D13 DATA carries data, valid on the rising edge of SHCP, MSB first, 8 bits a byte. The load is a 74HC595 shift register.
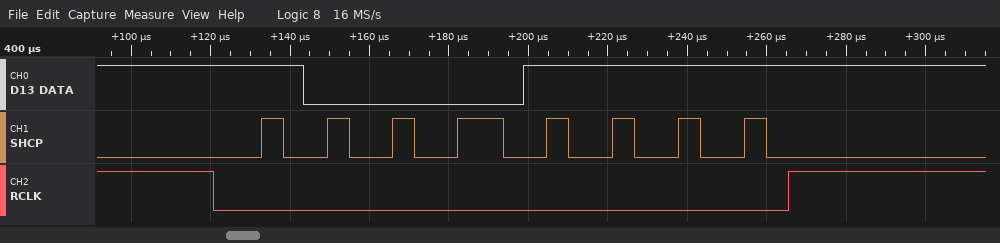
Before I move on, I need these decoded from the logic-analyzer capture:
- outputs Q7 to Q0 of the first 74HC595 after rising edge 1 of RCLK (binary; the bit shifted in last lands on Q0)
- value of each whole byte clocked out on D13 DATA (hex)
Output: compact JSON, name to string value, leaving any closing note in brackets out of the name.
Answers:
{"outputs Q7 to Q0 of the first 74HC595 after rising edge 1 of RCLK": "10001111", "value of each whole byte clocked out on D13 DATA": "0x8F"}
